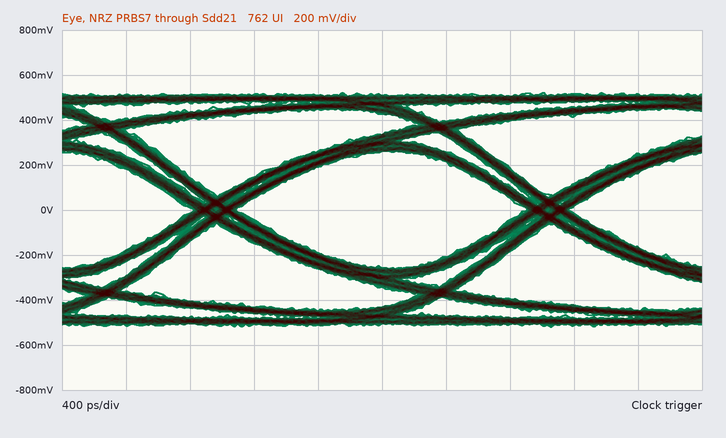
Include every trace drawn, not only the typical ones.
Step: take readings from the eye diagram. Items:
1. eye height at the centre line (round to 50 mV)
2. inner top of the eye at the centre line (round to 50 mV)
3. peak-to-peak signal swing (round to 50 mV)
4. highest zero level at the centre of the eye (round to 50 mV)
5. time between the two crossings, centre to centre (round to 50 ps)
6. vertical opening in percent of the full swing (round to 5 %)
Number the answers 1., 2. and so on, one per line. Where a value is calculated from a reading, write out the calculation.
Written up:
1. 500 mV
2. 250 mV
3. 1.05 V
4. -250 mV
5. 2.10 ns
6. 500 mV / 1.05 V ≈ 47.6 %, so 50 % to the nearest 5 %
